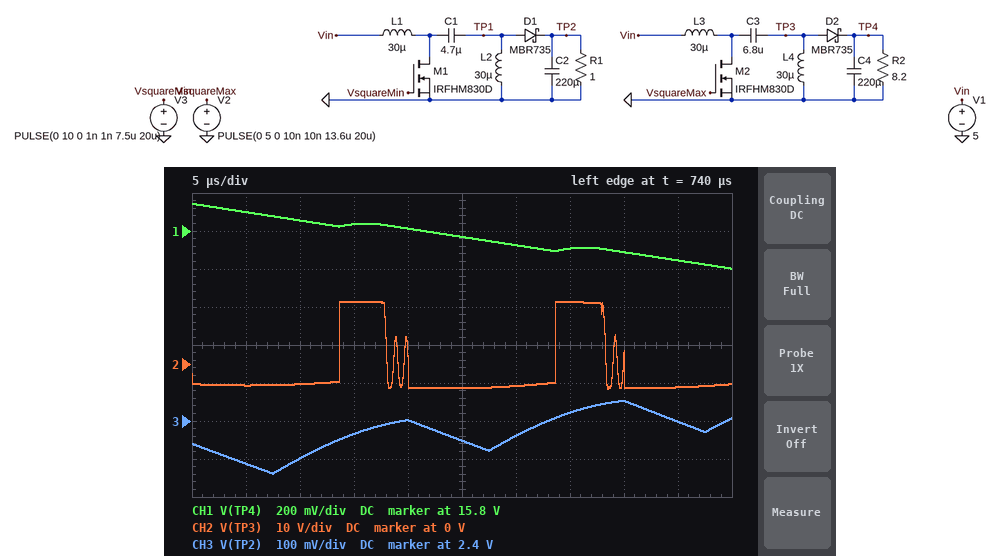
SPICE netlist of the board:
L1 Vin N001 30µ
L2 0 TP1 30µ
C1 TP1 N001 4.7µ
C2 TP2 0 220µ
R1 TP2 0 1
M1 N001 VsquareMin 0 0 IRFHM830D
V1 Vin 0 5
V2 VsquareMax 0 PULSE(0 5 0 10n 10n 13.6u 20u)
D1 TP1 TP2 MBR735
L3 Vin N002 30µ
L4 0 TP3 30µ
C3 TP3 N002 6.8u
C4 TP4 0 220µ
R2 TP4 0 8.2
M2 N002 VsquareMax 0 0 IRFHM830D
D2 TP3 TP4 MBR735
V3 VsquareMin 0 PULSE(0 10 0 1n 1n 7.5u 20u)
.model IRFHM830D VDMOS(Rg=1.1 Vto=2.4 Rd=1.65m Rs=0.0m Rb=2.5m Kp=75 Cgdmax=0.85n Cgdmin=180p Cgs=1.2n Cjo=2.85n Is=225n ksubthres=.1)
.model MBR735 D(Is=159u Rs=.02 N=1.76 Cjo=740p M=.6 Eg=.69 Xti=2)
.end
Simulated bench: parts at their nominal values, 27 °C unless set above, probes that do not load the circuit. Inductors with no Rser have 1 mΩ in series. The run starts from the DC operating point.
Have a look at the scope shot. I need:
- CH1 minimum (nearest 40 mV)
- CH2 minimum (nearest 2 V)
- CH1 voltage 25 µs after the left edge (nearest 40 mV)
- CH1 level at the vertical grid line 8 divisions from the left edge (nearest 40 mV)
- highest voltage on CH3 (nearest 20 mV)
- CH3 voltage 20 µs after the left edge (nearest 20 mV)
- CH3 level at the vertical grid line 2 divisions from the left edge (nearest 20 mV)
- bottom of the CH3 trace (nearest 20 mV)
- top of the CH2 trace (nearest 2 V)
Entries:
15.60 V
-6 V
15.76 V
15.68 V
2.46 V
2.40 V
2.30 V
2.26 V
16 V
